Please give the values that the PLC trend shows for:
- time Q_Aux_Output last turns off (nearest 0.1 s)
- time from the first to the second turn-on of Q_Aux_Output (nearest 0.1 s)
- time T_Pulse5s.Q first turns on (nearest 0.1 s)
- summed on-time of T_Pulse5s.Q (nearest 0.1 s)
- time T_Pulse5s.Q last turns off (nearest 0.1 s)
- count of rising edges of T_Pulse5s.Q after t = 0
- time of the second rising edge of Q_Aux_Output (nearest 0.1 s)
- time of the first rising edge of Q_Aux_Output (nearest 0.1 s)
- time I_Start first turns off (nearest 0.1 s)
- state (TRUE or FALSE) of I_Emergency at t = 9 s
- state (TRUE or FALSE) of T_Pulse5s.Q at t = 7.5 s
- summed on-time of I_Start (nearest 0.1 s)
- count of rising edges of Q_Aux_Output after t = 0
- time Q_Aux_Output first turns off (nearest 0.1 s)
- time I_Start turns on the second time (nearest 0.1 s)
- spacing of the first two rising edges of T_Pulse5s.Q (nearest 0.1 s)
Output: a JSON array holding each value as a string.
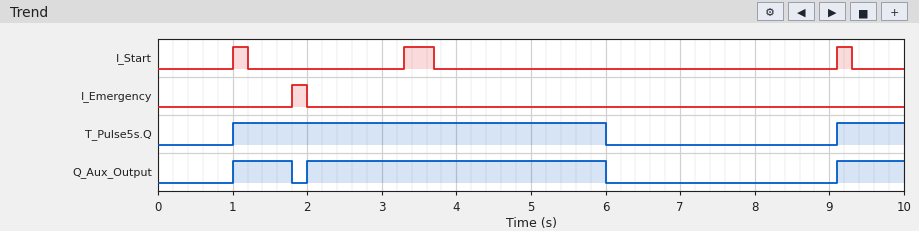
["6.0 s", "1.0 s", "1.0 s", "5.9 s", "6.0 s", "2", "2.0 s", "1.0 s", "1.2 s", "FALSE", "FALSE", "0.8 s", "3", "1.8 s", "3.3 s", "8.1 s"]
